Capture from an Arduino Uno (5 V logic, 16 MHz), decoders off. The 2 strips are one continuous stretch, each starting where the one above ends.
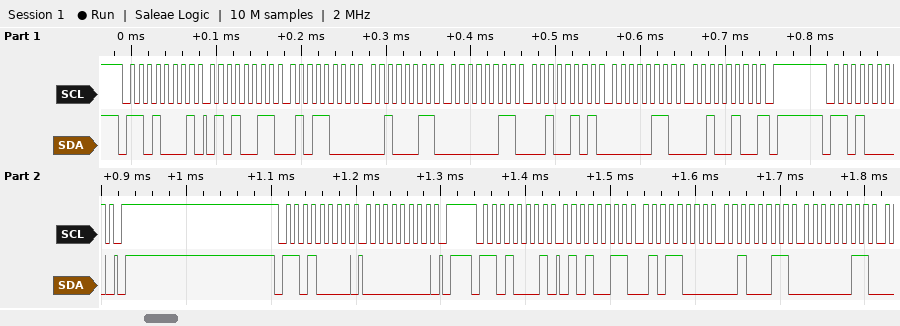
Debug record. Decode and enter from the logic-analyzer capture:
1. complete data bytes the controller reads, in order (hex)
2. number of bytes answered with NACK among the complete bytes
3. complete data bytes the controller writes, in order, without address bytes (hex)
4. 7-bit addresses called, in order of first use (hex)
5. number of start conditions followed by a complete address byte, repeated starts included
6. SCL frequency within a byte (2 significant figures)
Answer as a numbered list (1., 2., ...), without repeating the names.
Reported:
1. 53 58 23 03 25 06 24 53 58 23 03
2. 1
3. 00
4. 0x68
5. 4
6. 100 kHz
